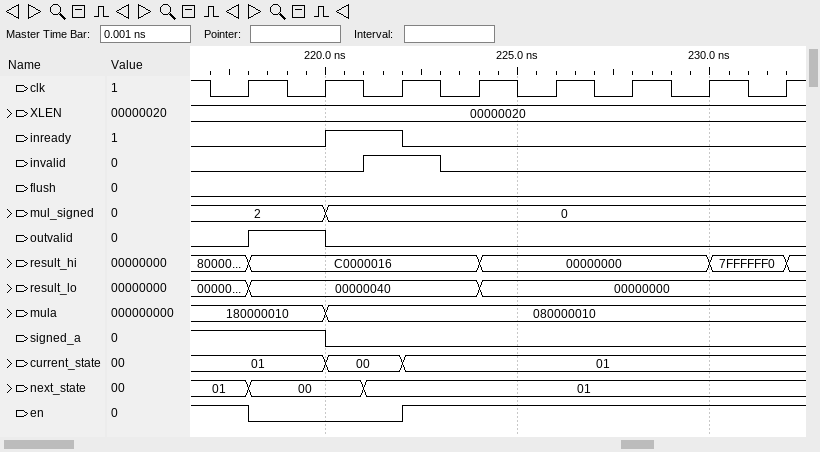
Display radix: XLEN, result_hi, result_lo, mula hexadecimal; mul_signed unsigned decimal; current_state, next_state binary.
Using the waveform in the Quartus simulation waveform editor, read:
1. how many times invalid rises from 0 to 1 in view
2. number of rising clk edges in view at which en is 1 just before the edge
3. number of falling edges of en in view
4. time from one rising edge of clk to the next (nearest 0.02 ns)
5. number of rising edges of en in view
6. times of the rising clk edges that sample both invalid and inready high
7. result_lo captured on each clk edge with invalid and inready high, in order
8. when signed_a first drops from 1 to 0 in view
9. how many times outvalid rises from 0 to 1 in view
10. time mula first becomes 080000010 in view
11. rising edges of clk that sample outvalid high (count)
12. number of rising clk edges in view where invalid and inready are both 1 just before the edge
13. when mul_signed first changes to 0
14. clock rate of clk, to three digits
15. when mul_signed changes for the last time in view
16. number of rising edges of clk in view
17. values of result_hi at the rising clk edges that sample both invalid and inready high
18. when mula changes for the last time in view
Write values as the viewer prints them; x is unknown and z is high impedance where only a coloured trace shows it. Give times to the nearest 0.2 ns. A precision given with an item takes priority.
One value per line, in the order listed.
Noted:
1
6
1
2 ns
1
222 ns
00000040
220 ns
1
220 ns
1
1
220 ns
500 MHz
220 ns
8
C0000016
220 ns
